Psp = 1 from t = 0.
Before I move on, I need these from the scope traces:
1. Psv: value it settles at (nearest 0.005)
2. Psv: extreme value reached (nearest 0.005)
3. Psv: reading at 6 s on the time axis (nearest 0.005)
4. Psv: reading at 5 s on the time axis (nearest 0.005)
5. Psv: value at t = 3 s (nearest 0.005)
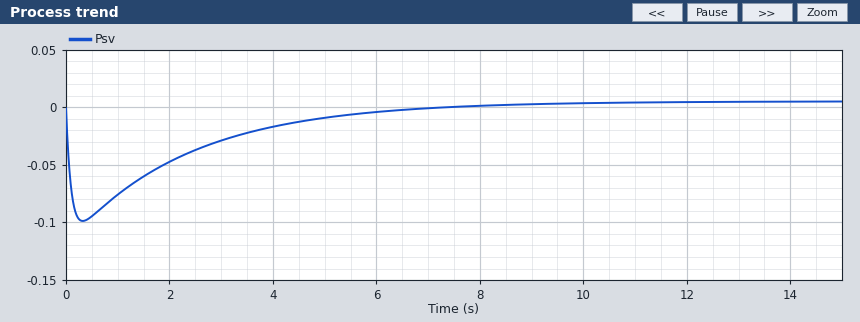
0.005
-0.100
-0.005
-0.010
-0.030
